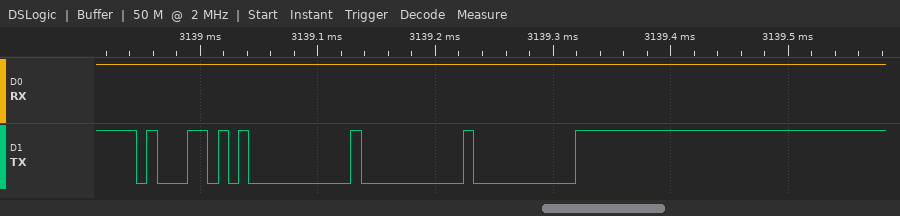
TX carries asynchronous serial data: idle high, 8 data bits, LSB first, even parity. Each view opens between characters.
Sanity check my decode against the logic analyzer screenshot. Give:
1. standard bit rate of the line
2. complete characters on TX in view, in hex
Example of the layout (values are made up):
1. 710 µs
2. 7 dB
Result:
1. 115200 baud
2. B1, 00, 00, 00
